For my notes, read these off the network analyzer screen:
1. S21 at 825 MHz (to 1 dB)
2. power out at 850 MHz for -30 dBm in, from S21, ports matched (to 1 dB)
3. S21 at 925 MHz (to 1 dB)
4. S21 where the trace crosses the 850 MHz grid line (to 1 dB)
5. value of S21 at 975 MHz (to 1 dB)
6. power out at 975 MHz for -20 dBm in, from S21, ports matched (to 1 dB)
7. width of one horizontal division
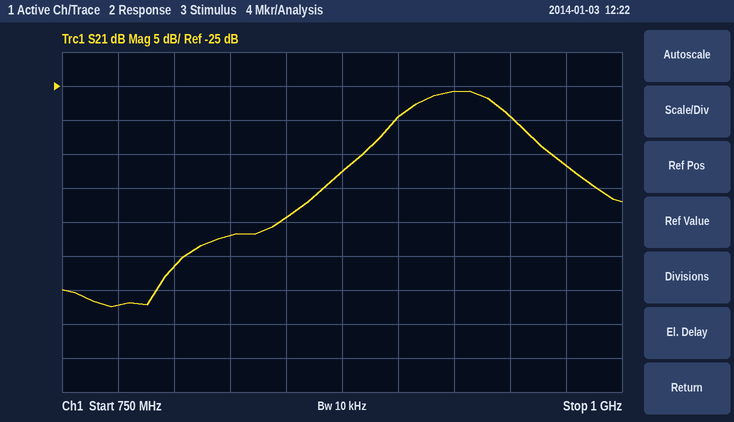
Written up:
-47 dB
-74 dBm
-26 dB
-44 dB
-37 dB
-57 dBm
25 MHz
